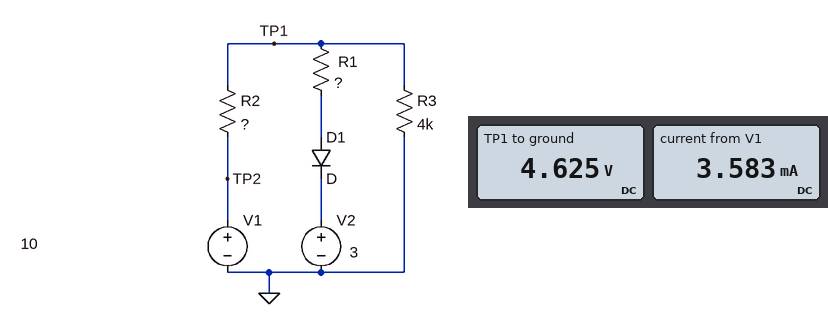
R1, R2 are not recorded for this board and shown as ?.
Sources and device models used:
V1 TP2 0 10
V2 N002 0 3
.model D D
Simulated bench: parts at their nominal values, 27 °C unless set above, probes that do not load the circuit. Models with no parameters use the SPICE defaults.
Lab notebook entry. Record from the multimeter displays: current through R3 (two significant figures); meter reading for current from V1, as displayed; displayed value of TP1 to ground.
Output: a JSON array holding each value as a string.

["1.2 mA", "3.583 mA", "4.625 V"]
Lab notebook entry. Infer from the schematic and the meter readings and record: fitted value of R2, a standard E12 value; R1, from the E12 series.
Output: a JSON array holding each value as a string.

["1.5 kΩ", "390 Ω"]
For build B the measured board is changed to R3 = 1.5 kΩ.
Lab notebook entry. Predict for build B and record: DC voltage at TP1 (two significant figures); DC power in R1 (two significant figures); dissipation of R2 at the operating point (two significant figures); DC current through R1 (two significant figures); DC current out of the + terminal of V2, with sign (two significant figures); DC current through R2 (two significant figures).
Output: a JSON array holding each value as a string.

["4.1 V", "540 µW", "23 mW", "1.2 mA", "-1.2 mA", "3.9 mA"]
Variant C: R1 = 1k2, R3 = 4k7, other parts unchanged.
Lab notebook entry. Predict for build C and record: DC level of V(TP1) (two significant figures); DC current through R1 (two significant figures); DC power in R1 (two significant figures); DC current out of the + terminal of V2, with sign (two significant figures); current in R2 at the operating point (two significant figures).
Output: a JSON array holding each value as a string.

["5.7 V", "1.7 mA", "3.4 mW", "-1.7 mA", "2.9 mA"]
